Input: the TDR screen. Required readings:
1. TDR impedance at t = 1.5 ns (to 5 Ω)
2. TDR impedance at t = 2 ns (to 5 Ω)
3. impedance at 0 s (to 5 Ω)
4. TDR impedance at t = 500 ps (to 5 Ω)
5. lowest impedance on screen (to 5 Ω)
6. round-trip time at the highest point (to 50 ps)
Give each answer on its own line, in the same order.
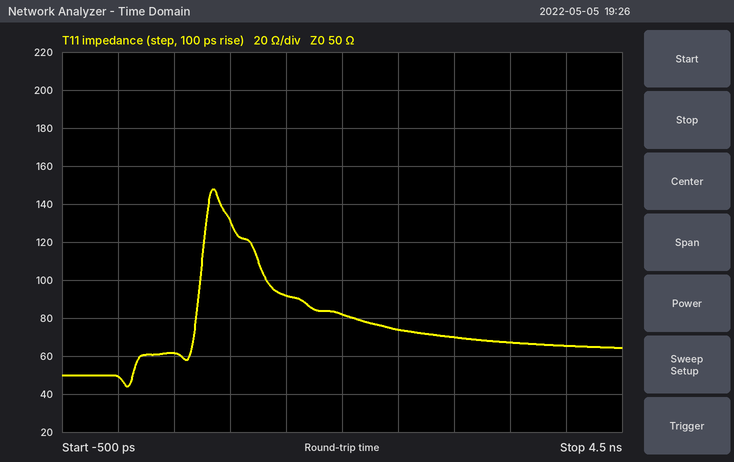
90 Ω
80 Ω
50 Ω
60 Ω
45 Ω
850 ps
